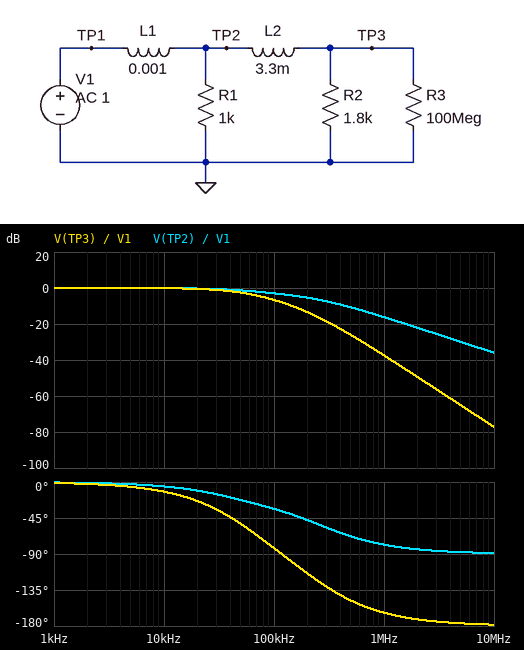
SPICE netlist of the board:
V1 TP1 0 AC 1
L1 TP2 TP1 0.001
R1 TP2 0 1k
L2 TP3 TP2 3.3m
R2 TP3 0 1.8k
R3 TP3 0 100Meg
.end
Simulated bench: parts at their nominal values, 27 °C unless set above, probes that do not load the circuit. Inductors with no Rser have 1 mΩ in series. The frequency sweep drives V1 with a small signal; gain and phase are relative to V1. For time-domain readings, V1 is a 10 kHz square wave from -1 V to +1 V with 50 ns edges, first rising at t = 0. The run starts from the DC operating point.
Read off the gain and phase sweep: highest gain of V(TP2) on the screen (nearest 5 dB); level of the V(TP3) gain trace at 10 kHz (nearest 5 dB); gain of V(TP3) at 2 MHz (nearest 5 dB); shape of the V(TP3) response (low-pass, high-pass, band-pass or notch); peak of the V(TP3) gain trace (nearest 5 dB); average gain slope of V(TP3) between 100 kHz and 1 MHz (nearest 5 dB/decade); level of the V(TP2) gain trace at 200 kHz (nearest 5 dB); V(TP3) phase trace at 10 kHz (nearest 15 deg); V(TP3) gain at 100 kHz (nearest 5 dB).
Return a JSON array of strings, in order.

["0 dB", "0 dB", "-50 dB", "low-pass", "0 dB", "-30 dB/decade", "-5 dB", "-15 deg", "-5 dB"]
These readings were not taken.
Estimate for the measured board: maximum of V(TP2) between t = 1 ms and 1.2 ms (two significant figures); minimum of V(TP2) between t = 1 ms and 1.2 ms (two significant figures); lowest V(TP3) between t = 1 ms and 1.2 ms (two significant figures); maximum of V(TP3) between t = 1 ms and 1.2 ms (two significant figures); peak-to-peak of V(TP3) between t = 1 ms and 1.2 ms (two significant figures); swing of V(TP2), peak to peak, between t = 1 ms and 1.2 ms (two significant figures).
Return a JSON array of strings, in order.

["1.0 V", "-1.0 V", "-1.0 V", "1.0 V", "2.0 V", "2.0 V"]
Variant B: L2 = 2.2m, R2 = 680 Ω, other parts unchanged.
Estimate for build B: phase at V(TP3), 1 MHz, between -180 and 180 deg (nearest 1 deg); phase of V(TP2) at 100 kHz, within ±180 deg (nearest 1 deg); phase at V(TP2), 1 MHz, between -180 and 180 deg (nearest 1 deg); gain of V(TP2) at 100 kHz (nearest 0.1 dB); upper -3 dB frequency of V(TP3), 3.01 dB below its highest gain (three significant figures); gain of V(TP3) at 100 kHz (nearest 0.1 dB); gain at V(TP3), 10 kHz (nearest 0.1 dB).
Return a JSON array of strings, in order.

["-164 deg", "-31 deg", "-77 deg", "-4.0 dB", "30.9 kHz", "-11.1 dB", "-0.4 dB"]
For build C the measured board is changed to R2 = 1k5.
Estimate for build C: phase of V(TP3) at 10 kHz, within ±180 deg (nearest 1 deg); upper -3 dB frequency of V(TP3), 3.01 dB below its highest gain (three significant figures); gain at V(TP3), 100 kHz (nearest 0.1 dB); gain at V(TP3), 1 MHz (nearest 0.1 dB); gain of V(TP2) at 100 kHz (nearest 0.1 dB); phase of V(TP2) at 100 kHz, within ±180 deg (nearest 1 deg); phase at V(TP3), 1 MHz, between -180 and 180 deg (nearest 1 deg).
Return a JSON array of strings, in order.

["-14 deg", "48.0 kHz", "-7.7 dB", "-39.0 dB", "-3.1 dB", "-33 deg", "-164 deg"]
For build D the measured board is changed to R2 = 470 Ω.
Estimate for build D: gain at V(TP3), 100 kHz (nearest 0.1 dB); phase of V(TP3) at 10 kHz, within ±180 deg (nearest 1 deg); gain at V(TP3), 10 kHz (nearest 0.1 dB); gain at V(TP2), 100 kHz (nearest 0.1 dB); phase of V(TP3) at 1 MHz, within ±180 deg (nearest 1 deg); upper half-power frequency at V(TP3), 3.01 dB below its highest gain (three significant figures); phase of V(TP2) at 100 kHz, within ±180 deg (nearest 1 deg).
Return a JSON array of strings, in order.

["-16.4 dB", "-33 deg", "-1.3 dB", "-3.3 dB", "-167 deg", "16.8 kHz", "-28 deg"]
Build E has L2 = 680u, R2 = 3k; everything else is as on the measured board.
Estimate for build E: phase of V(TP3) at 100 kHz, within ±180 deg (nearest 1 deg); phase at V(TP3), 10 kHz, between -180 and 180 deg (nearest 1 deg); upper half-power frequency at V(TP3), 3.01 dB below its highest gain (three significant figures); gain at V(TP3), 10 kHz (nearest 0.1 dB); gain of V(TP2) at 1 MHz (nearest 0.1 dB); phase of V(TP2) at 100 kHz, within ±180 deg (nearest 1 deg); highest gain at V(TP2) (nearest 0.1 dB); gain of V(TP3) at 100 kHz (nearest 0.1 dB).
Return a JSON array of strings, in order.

["-47 deg", "-6 deg", "112 kHz", "0 dB", "-17.2 dB", "-39 deg", "0 dB", "-2.5 dB"]
